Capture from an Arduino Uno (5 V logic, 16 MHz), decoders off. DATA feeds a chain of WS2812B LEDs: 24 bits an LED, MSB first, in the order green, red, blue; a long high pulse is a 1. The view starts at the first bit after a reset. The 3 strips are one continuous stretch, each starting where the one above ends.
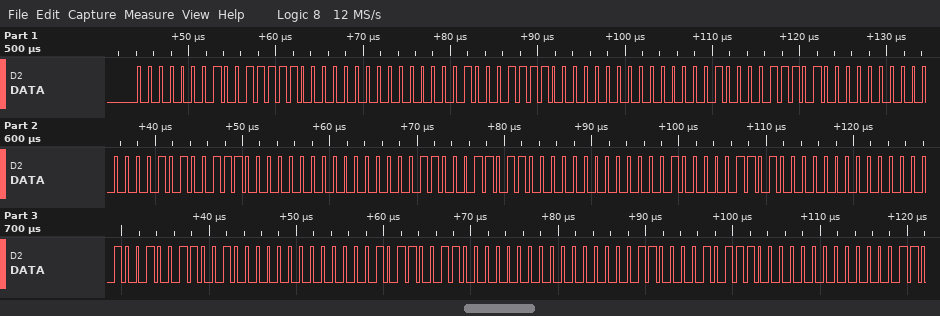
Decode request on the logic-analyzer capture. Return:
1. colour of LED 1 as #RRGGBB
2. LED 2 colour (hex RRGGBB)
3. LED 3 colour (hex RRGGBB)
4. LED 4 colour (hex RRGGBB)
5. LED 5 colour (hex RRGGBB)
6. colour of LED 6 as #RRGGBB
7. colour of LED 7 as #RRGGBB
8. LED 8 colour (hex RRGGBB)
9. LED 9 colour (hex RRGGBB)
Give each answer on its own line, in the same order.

#3E0100
#3C0200
#3A0400
#380500
#360600
#340800
#320900
#300B00
#2E0C00
